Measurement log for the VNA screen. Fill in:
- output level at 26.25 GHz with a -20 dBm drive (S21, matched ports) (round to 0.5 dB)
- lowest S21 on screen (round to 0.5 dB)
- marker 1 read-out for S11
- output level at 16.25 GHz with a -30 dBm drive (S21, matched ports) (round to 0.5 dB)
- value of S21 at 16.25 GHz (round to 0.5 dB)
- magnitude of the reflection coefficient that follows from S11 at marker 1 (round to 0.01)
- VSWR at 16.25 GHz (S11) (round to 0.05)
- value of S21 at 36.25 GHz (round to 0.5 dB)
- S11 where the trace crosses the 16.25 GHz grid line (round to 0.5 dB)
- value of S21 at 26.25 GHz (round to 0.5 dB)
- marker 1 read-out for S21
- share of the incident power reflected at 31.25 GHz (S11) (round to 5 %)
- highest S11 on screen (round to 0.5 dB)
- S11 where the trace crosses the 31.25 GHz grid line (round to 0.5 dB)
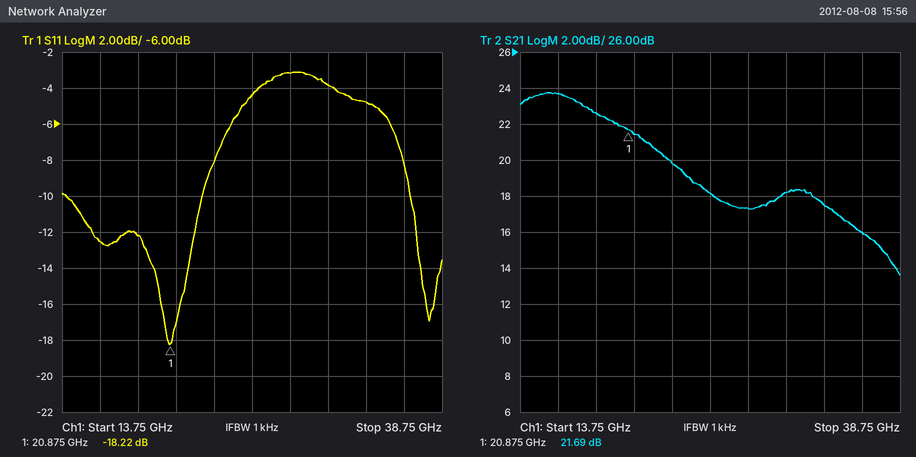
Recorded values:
-2.0 dBm
13.5 dB
-18.22 dB
-6.5 dBm
23.5 dB
0.12
1.60
16.0 dB
-12.5 dB
18.0 dB
21.69 dB
40 %
-3.0 dB
-4.0 dB
